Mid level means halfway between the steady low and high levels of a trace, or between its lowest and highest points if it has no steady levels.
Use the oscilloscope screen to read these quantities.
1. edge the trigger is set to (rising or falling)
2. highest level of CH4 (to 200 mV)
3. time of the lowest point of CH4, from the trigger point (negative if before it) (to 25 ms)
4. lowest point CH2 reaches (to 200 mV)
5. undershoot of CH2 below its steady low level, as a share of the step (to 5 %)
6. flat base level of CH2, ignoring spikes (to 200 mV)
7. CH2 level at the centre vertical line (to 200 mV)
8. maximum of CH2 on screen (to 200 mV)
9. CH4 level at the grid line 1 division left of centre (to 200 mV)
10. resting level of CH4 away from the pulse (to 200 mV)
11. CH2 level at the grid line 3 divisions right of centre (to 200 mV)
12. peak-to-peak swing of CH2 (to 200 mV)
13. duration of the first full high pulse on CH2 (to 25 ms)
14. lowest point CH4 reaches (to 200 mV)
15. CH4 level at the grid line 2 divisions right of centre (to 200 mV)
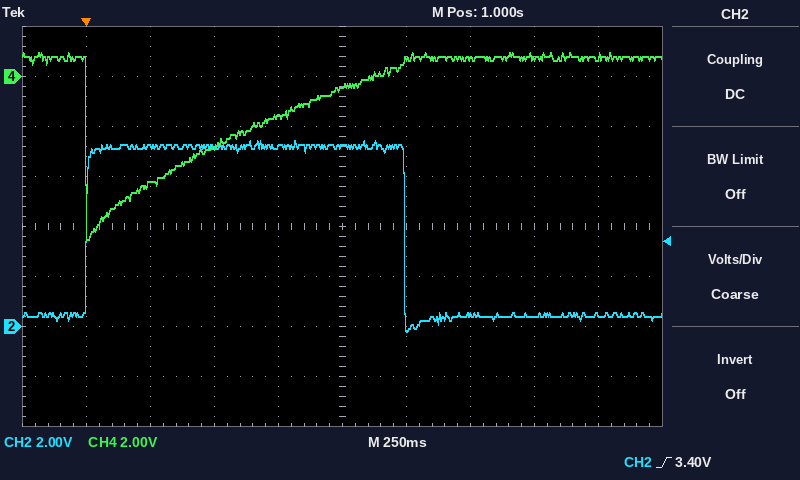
rising
1.0 V
0 ms
-200 mV
10 %
400 mV
7.2 V
7.4 V
-1.6 V
800 mV
400 mV
7.6 V
1.250 s
-6.6 V
800 mV
